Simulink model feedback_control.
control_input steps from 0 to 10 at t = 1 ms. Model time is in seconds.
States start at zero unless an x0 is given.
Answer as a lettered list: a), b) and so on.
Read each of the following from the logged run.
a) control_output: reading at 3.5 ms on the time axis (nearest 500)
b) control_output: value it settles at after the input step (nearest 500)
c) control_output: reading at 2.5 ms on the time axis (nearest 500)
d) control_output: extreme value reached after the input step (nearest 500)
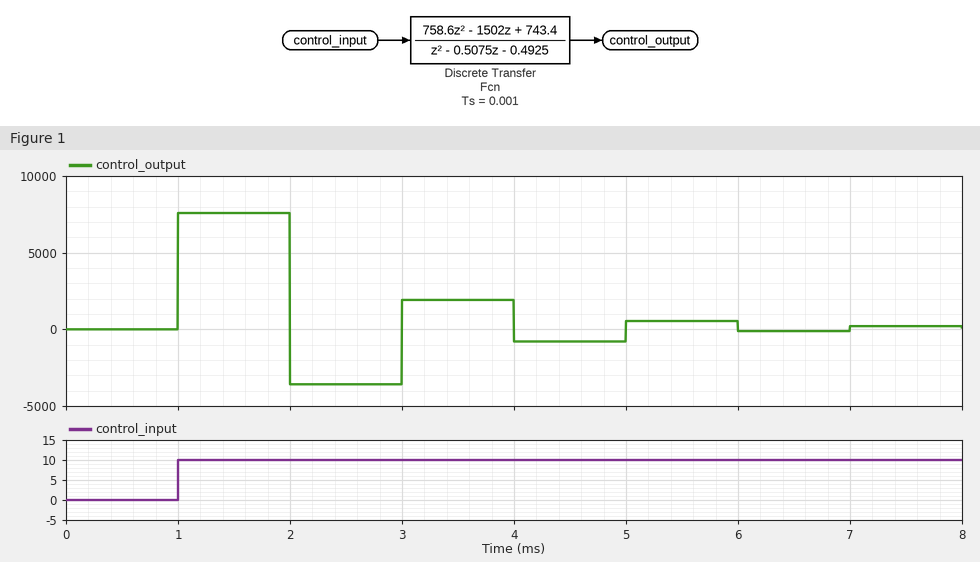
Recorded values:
a) 2000
b) 0
c) -3500
d) 7500
